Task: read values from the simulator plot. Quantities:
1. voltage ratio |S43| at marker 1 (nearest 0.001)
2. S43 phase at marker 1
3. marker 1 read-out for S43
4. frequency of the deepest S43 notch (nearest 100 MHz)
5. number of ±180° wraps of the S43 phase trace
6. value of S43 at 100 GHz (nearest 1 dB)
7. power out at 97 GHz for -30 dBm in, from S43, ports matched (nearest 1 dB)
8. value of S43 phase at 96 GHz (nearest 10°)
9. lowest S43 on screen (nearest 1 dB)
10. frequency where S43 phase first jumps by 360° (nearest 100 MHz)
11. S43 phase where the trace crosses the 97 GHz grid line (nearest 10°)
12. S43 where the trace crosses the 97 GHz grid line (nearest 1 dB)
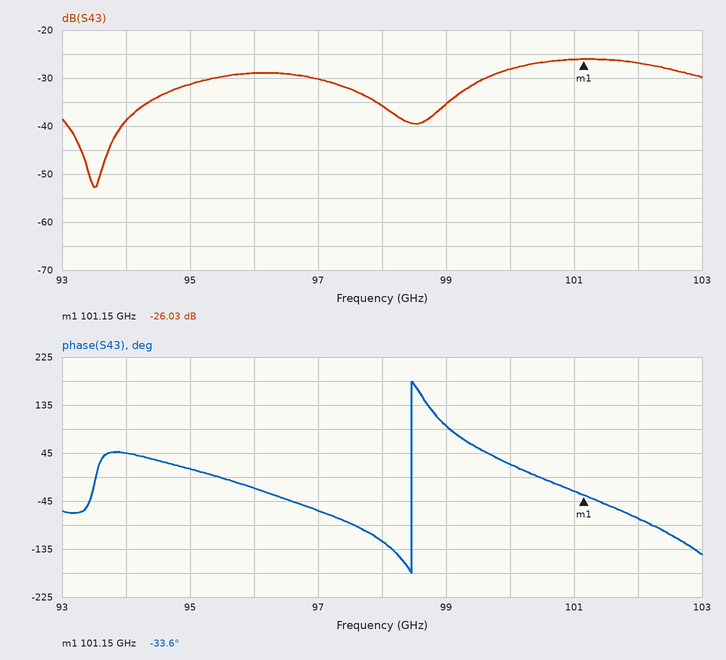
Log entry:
0.050
-33.6°
-26.03 dB
93.5 GHz
1
-28 dB
-60 dBm
-20°
-53 dB
98.5 GHz
-60°
-30 dB
